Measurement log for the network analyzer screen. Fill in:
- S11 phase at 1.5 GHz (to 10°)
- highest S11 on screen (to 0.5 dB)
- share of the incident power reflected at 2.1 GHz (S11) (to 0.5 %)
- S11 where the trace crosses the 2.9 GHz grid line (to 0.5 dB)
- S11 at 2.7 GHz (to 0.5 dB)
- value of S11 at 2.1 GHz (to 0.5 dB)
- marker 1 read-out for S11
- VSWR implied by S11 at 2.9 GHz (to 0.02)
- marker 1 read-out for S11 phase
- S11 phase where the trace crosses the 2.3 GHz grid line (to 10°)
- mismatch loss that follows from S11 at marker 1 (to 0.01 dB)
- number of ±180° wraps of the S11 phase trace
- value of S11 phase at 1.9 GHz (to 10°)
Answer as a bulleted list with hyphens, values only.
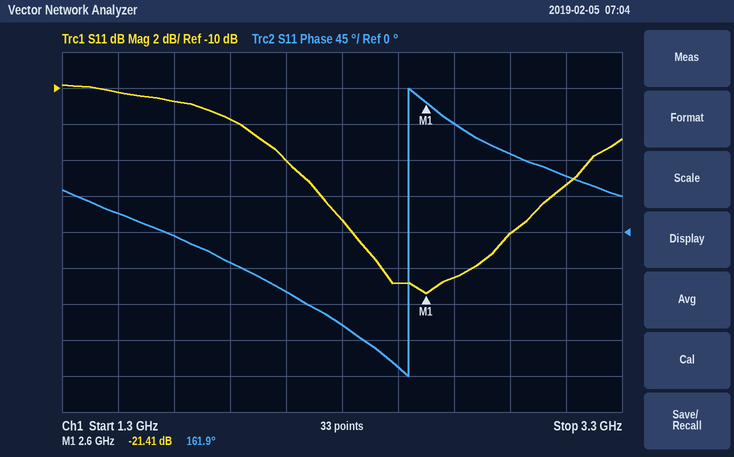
- 20°
- -10.0 dB
- 4.0 %
- -18.0 dB
- -20.5 dB
- -14.0 dB
- -21.41 dB
- 1.28
- 161.9°
- -120°
- 0.03 dB
- 1
- -40°
